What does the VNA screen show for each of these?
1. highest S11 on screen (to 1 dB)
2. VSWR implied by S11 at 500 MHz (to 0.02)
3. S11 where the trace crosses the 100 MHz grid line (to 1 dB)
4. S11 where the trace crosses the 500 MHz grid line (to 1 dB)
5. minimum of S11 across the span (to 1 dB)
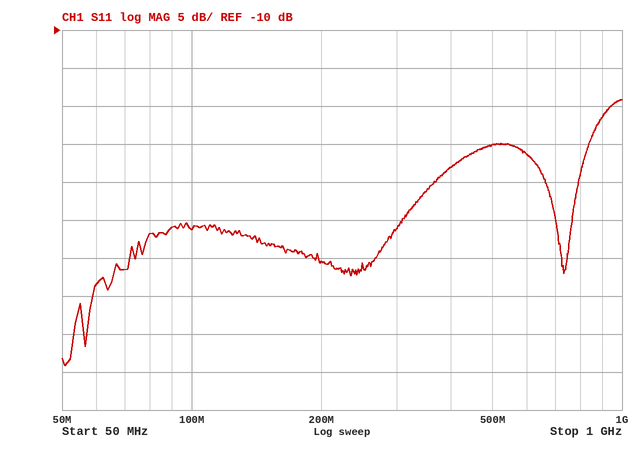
-19 dB
1.12
-36 dB
-25 dB
-54 dB
